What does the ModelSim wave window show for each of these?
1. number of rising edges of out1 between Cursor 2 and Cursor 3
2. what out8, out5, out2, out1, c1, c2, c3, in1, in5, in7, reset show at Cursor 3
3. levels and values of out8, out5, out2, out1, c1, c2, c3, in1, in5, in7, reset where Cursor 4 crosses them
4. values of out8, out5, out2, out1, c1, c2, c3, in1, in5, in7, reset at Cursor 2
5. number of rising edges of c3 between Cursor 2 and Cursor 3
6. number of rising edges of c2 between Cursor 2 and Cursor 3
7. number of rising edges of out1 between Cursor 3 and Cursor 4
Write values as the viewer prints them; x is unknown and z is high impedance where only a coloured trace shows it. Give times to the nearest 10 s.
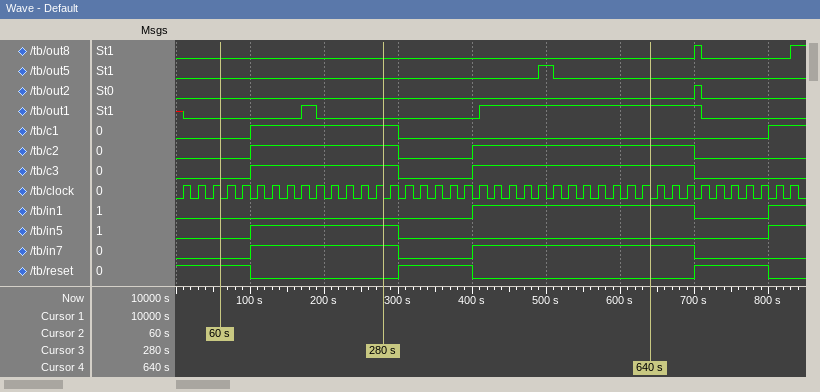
1
out8=0, out5=0, out2=0, out1=0, c1=1, c2=1, c3=1, in1=0, in5=1, in7=1, reset=0
out8=0, out5=0, out2=0, out1=1, c1=0, c2=1, c3=1, in1=1, in5=0, in7=1, reset=0
out8=0, out5=0, out2=0, out1=0, c1=0, c2=0, c3=0, in1=0, in5=0, in7=0, reset=1
1
1
1
